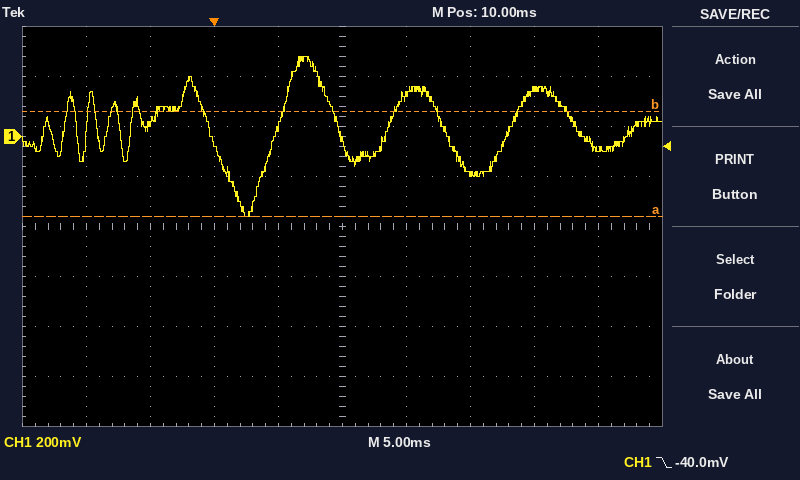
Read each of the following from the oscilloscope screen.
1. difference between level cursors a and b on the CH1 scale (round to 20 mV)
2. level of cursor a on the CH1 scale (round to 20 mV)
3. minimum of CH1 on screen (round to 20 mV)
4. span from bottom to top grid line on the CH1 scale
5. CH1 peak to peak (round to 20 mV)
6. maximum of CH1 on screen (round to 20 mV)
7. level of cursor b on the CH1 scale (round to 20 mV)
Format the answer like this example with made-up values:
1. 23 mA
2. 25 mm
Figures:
1. 420 mV
2. -320 mV
3. -320 mV
4. 1.6 V
5. 640 mV
6. 320 mV
7. 100 mV
